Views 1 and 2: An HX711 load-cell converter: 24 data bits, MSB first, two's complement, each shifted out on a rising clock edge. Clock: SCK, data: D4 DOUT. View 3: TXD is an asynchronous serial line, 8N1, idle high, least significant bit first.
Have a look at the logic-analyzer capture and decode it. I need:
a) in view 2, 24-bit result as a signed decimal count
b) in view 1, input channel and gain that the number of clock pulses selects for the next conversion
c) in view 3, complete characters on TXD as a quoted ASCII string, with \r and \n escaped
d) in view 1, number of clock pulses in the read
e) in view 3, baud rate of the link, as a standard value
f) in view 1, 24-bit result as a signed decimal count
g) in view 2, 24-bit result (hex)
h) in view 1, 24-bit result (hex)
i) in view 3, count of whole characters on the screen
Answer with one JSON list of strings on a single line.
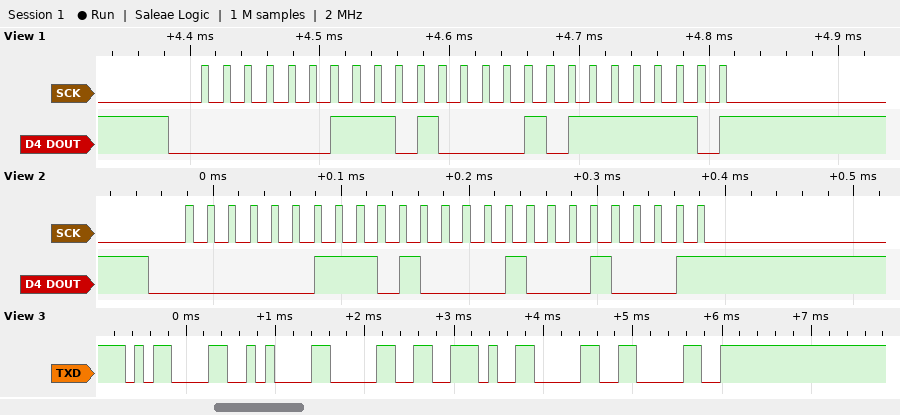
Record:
["237841", "channel A, gain 128", "\"\\r\\n0.00\"", "25", "9600 baud", "237950", "0x03A111", "0x03A17E", "6"]
